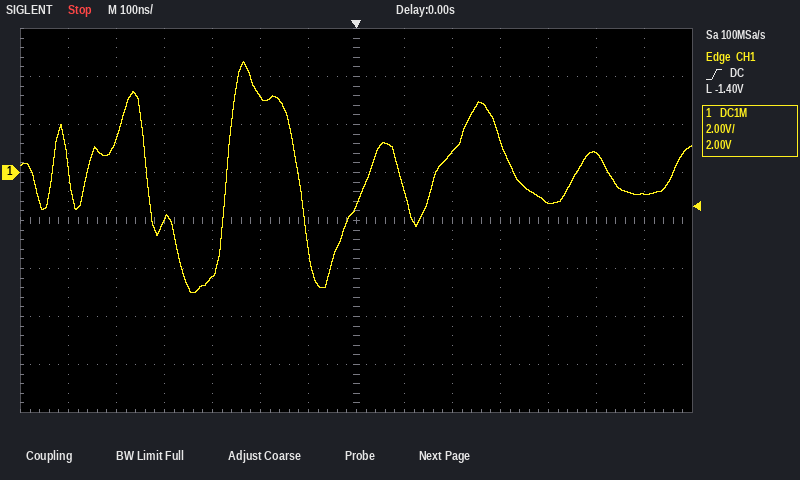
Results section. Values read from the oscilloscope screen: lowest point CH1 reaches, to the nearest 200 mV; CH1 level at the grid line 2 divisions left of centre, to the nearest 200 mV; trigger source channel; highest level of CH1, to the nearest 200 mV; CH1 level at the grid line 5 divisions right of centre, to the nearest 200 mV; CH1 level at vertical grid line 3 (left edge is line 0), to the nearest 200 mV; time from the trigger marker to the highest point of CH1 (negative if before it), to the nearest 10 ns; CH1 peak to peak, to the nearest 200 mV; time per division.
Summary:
-5.0 V
3.2 V
CH1
4.6 V
800 mV
-2.0 V
-230 ns
9.6 V
100 ns
